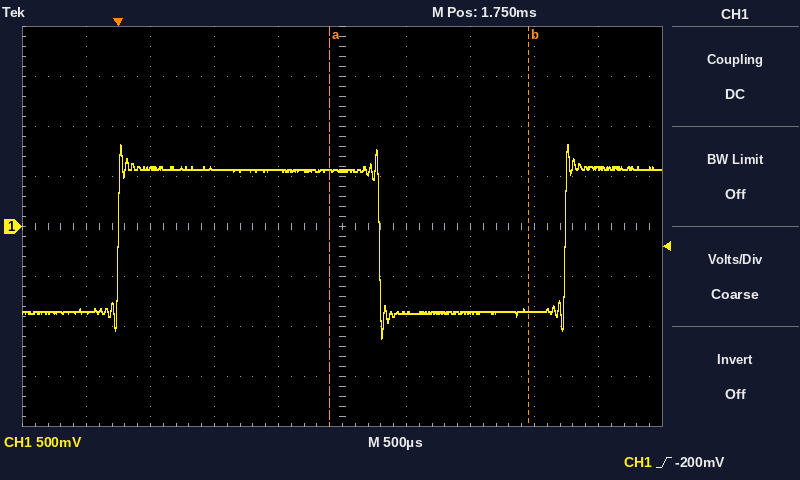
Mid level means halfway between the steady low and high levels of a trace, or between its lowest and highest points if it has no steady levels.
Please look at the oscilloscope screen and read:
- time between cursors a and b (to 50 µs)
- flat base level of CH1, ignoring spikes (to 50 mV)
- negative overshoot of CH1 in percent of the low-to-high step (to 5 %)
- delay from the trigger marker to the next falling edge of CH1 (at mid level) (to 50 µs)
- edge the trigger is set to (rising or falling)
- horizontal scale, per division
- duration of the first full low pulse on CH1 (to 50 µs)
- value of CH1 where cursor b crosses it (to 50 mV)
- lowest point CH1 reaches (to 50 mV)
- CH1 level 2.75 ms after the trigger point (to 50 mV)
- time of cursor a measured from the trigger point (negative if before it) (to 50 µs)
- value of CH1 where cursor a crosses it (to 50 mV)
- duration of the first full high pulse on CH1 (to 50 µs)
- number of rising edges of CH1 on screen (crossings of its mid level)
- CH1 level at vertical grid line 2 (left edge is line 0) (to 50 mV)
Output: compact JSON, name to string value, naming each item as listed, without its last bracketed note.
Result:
{"time between cursors a and b": "1.55 ms", "flat base level of CH1, ignoring spikes": "-850 mV", "negative overshoot of CH1 in percent of the low-to-high step": "20 %", "delay from the trigger marker to the next falling edge of CH1 (at mid level)": "2.05 ms", "edge the trigger is set to": "rising", "horizontal scale, per division": "500 µs", "duration of the first full low pulse on CH1": "1.45 ms", "value of CH1 where cursor b crosses it": "-850 mV", "lowest point CH1 reaches": "-1.10 V", "CH1 level 2.75 ms after the trigger point": "-850 mV", "time of cursor a measured from the trigger point (negative if before it)": "+1.65 ms", "value of CH1 where cursor a crosses it": "550 mV", "duration of the first full high pulse on CH1": "2.05 ms", "number of rising edges of CH1 on screen": "2", "CH1 level at vertical grid line 2 (left edge is line 0)": "600 mV"}
